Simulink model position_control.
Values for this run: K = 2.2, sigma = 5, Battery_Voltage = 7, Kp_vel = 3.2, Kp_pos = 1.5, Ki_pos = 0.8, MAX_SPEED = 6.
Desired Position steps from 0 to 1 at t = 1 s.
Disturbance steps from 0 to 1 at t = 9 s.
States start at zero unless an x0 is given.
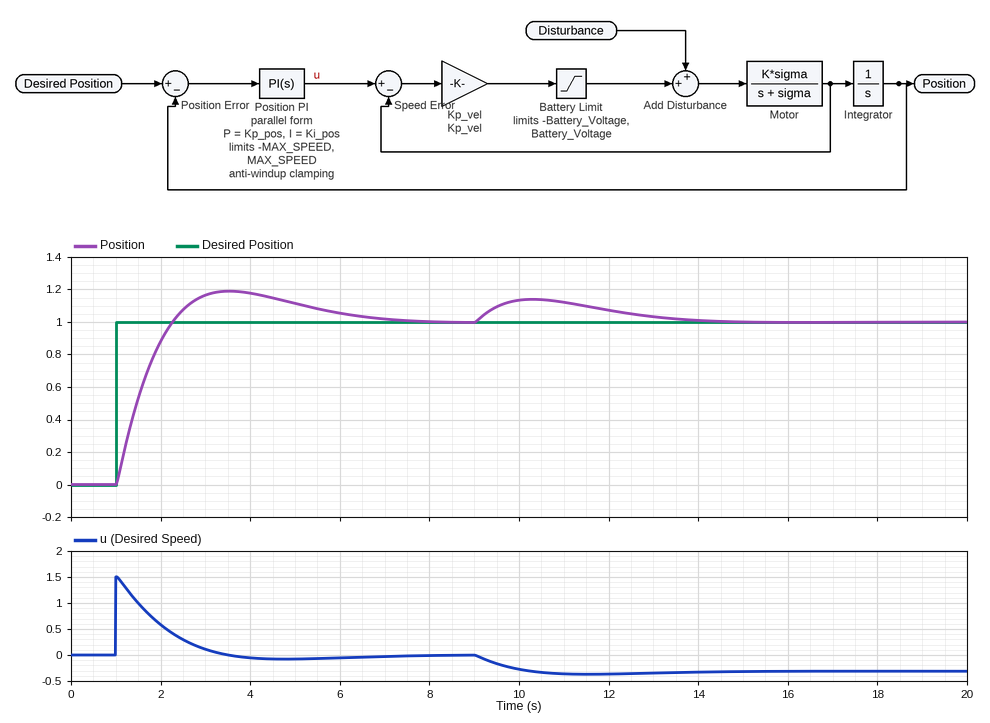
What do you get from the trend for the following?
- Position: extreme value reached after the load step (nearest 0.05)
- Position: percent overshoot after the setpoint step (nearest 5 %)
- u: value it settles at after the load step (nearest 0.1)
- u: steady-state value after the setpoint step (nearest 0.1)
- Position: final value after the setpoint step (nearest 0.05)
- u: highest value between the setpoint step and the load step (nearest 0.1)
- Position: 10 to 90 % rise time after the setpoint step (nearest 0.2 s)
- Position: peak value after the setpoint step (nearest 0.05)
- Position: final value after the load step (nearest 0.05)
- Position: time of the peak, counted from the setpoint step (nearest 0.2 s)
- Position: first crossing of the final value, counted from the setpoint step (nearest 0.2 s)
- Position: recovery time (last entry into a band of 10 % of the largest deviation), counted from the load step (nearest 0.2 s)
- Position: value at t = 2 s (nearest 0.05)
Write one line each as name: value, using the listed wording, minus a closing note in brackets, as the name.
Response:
Position: extreme value reached after the load step: 1.15
Position: percent overshoot after the setpoint step: 20 %
u: value it settles at after the load step: -0.3
u: steady-state value after the setpoint step: 0.0
Position: final value after the setpoint step: 1.00
u: highest value between the setpoint step and the load step: 1.5
Position: 10 to 90 % rise time after the setpoint step: 1.0 s
Position: peak value after the setpoint step: 1.20
Position: final value after the load step: 1.00
Position: time of the peak, counted from the setpoint step: 2.6 s
Position: first crossing of the final value, counted from the setpoint step: 1.2 s
Position: recovery time (last entry into a band of 10 % of the largest deviation), counted from the load step: 4.8 s
Position: value at t = 2 s: 0.90
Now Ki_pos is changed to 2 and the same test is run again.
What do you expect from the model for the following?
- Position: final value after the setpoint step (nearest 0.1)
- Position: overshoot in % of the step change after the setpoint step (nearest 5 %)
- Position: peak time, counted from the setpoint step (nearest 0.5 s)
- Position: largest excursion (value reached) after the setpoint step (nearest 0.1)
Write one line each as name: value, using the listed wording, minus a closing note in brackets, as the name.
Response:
Position: final value after the setpoint step: 1.0
Position: overshoot in % of the step change after the setpoint step: 30 %
Position: peak time, counted from the setpoint step: 2.0 s
Position: largest excursion (value reached) after the setpoint step: 1.3
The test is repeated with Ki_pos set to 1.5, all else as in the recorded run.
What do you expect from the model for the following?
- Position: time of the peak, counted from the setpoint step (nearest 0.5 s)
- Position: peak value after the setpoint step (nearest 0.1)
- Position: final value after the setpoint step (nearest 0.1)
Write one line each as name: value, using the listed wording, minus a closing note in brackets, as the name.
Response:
Position: time of the peak, counted from the setpoint step: 2.0 s
Position: peak value after the setpoint step: 1.3
Position: final value after the setpoint step: 1.0
